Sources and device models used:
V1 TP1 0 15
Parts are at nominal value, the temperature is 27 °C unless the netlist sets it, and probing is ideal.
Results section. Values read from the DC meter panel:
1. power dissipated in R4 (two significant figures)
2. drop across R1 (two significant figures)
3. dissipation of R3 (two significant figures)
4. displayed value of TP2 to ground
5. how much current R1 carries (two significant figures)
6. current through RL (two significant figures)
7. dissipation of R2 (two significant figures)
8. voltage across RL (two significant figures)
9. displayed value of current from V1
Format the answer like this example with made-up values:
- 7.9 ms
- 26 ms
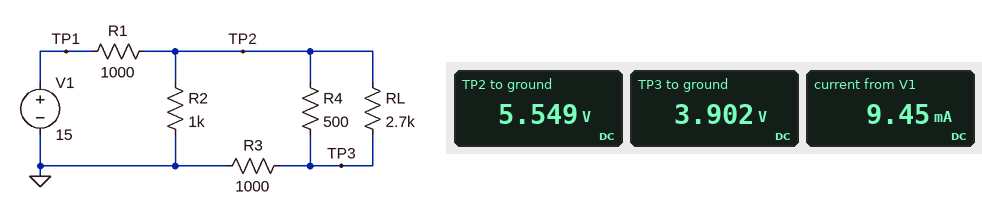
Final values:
- 5.4 mW
- 9.5 V
- 15 mW
- 5.549 V
- 9.5 mA
- 610 µA
- 31 mW
- 1.6 V
- 9.45 mA
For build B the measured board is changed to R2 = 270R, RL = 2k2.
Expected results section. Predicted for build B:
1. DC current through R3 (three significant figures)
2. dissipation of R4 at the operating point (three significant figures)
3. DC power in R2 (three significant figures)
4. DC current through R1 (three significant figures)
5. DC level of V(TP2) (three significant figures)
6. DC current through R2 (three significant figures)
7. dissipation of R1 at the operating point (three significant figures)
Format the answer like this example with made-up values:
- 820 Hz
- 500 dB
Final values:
- 1.97 mA
- 1.29 mW
- 28.4 mW
- 12.2 mA
- 2.77 V
- 10.3 mA
- 150 mW
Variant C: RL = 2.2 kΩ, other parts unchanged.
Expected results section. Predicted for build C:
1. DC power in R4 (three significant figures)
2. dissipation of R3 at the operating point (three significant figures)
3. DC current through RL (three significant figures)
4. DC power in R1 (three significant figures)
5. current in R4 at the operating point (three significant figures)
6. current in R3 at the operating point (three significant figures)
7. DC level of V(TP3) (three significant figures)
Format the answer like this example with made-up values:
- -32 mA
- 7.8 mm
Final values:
- 5.13 mW
- 15.5 mW
- 728 µA
- 89.6 mW
- 3.20 mA
- 3.93 mA
- 3.93 V
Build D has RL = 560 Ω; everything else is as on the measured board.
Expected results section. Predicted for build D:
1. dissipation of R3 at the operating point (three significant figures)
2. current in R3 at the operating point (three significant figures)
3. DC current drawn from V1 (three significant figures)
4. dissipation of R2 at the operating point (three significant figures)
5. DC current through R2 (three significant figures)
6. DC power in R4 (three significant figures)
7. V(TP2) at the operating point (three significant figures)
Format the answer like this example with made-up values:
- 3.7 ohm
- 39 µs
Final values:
- 18.1 mW
- 4.25 mA
- 9.63 mA
- 28.9 mW
- 5.37 mA
- 2.52 mW
- 5.37 V
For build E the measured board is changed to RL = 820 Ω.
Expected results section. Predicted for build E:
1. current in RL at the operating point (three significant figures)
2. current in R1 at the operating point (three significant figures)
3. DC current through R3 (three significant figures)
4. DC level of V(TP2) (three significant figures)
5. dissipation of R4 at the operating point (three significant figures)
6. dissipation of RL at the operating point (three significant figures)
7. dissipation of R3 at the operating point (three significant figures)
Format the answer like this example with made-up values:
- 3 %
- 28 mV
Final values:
- 1.57 mA
- 9.57 mA
- 4.14 mA
- 5.43 V
- 3.31 mW
- 2.02 mW
- 17.2 mW
